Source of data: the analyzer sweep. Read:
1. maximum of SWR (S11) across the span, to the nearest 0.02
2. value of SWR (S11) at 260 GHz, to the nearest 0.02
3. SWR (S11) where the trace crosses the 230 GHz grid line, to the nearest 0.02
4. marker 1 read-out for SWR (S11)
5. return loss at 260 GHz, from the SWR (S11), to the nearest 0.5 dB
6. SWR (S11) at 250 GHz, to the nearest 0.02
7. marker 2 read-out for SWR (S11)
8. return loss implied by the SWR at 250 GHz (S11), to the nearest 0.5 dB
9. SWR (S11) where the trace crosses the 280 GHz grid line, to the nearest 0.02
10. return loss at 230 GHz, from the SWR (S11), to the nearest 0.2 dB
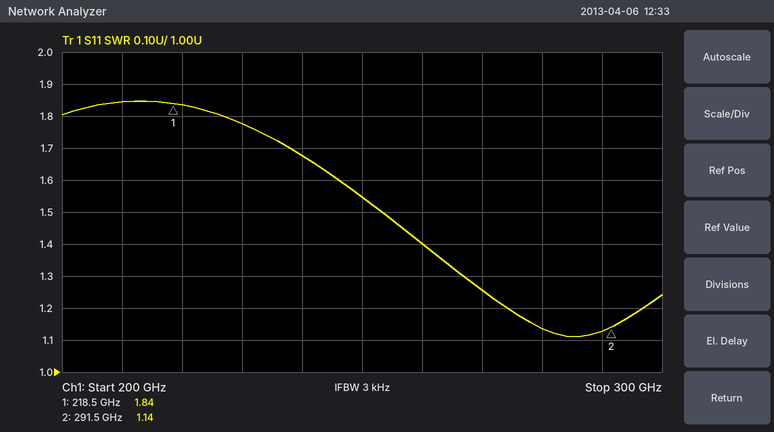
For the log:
1.84
1.40
1.78
1.84
15.5 dB
1.54
1.14
13.5 dB
1.14
11.0 dB
